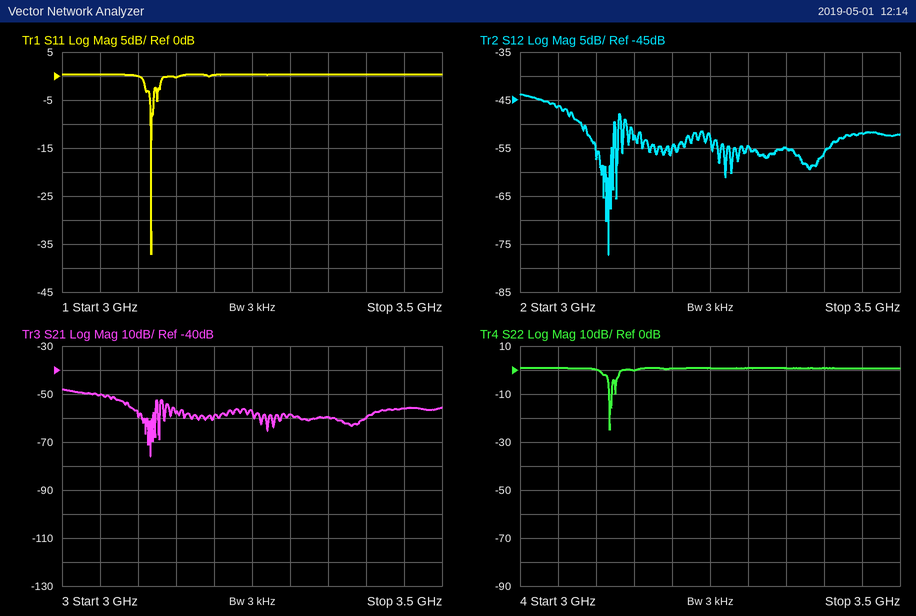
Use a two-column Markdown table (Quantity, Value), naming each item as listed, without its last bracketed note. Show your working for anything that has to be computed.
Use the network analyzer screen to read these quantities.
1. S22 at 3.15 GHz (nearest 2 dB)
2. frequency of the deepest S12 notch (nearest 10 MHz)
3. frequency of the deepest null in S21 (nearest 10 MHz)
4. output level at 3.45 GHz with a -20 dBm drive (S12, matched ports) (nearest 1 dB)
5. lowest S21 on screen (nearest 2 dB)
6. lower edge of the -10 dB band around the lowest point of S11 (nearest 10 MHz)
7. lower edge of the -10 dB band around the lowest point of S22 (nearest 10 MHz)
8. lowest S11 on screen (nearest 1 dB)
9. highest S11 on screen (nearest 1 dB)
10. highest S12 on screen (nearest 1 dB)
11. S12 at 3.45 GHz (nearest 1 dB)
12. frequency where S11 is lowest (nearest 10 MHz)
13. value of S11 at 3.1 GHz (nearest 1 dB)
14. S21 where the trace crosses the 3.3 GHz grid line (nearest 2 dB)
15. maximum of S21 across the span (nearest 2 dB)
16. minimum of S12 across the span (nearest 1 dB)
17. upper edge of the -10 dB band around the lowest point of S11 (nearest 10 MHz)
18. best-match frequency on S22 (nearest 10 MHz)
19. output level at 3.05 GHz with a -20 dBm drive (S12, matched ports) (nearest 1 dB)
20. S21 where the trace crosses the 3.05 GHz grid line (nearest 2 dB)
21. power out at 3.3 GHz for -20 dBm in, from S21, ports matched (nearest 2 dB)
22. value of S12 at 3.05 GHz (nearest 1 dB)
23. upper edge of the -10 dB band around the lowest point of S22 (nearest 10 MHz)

| Quantity | Value |
|---|---|
| S22 at 3.15 GHz | 0 dB |
| frequency of the deepest S12 notch | 3.12 GHz |
| frequency of the deepest null in S21 | 3.12 GHz |
| output level at 3.45 GHz with a -20 dBm drive (S12, matched ports) | -20 dBm + (-52 dB) = -72 dBm |
| lowest S21 on screen | -76 dB |
| lower edge of the -10 dB band around the lowest point of S11 | 3.12 GHz |
| lower edge of the -10 dB band around the lowest point of S22 | 3.12 GHz |
| lowest S11 on screen | -37 dB |
| highest S11 on screen | 0 dB |
| highest S12 on screen | -44 dB |
| S12 at 3.45 GHz | -52 dB |
| frequency where S11 is lowest | 3.12 GHz |
| value of S11 at 3.1 GHz | 0 dB |
| S21 where the trace crosses the 3.3 GHz grid line | -58 dB |
| maximum of S21 across the span | -48 dB |
| minimum of S12 across the span | -77 dB |
| upper edge of the -10 dB band around the lowest point of S11 | 3.12 GHz |
| best-match frequency on S22 | 3.12 GHz |
| output level at 3.05 GHz with a -20 dBm drive (S12, matched ports) | -20 dBm + (-46 dB) = -66 dBm |
| S21 where the trace crosses the 3.05 GHz grid line | -50 dB |
| power out at 3.3 GHz for -20 dBm in, from S21, ports matched | -20 dBm + (-58 dB) = -78 dBm |
| value of S12 at 3.05 GHz | -46 dB |
| upper edge of the -10 dB band around the lowest point of S22 | 3.12 GHz |
